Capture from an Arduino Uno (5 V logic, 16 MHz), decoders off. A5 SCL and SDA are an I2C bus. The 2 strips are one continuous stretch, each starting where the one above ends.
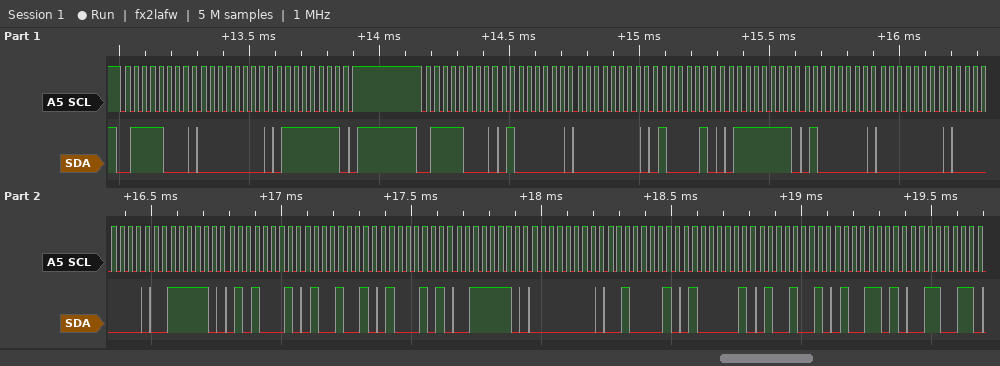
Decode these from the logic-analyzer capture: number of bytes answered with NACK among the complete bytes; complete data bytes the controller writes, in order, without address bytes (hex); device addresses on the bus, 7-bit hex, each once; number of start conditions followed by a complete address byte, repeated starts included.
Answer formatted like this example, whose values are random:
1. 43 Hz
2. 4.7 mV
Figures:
1. 0
2. 00 7F 40 00 42 7F 40 00 00 3E 51 49 45 3E 00 21 41 49 4D 33
3. 0x3C
4. 2
